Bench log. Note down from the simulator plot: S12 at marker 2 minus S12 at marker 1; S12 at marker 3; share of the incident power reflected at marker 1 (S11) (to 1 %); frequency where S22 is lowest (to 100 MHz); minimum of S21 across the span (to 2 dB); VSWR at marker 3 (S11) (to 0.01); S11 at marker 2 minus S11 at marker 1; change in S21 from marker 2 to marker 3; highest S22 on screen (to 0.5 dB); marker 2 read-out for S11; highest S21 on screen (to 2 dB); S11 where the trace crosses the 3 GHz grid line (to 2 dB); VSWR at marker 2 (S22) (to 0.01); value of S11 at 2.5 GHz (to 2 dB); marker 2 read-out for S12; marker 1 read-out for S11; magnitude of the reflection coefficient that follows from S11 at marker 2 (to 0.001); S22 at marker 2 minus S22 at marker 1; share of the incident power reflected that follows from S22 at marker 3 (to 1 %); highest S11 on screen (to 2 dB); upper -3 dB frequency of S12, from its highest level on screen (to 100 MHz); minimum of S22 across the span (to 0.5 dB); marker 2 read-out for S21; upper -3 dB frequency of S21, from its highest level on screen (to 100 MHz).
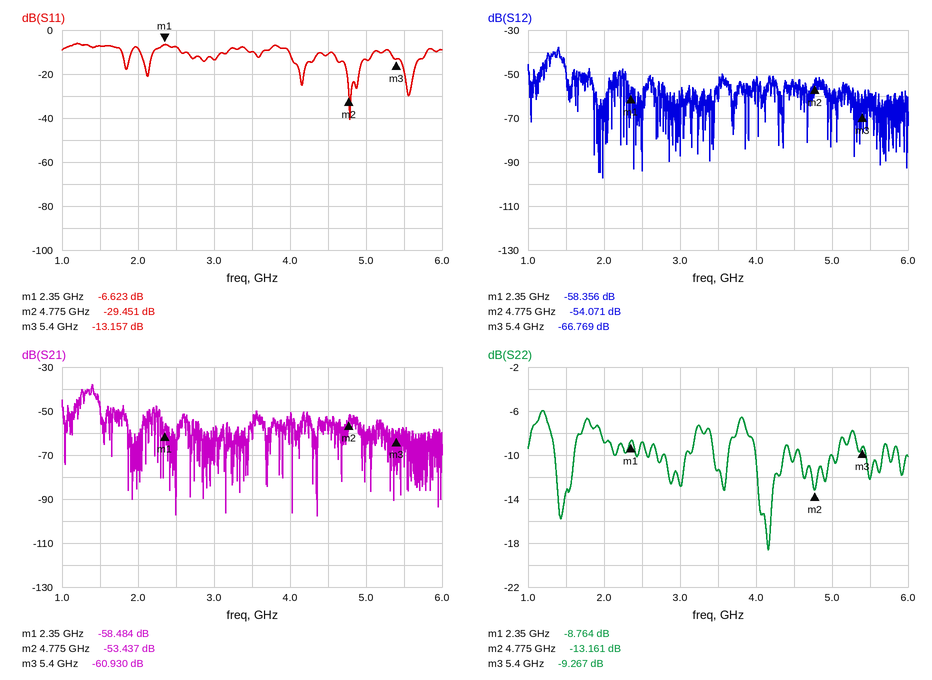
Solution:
4.285 dB
-66.769 dB
22 %
4.2 GHz
-98 dB
1.56
-22.828 dB
-7.493 dB
-6.0 dB
-29.451 dB
-38 dB
-14 dB
1.56
-8 dB
-54.071 dB
-6.623 dB
0.034
-4.397 dB
12 %
-6 dB
1.4 GHz
-18.5 dB
-53.437 dB
1.4 GHz
